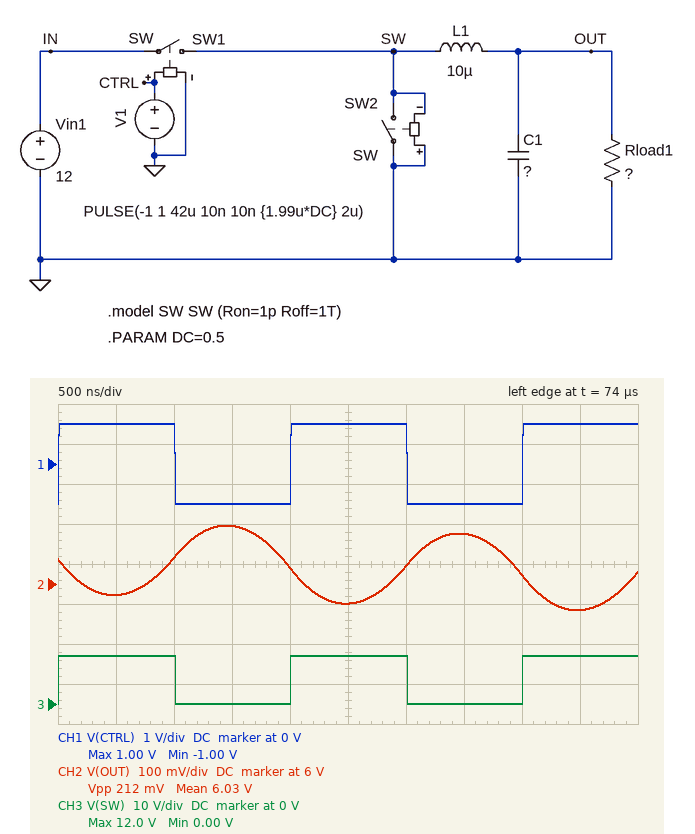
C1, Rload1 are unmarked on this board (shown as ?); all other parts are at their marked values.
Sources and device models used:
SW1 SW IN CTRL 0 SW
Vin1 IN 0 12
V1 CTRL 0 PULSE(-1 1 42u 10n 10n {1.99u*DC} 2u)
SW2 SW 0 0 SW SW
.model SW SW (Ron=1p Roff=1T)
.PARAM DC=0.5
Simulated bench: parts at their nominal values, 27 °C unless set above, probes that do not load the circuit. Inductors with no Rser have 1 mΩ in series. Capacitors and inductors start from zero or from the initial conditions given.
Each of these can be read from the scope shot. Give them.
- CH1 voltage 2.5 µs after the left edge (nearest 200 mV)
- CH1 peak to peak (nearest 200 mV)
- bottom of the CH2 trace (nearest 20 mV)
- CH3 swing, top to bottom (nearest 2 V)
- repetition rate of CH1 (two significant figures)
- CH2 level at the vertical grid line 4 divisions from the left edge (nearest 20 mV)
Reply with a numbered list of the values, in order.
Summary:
1. 1.0 V
2. 2.0 V
3. 5.94 V
4. 12 V
5. 500 kHz
6. 6.04 V
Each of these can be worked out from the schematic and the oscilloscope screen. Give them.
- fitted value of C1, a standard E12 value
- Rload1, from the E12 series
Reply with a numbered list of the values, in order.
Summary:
1. 820 nF
2. 3.9 Ω
